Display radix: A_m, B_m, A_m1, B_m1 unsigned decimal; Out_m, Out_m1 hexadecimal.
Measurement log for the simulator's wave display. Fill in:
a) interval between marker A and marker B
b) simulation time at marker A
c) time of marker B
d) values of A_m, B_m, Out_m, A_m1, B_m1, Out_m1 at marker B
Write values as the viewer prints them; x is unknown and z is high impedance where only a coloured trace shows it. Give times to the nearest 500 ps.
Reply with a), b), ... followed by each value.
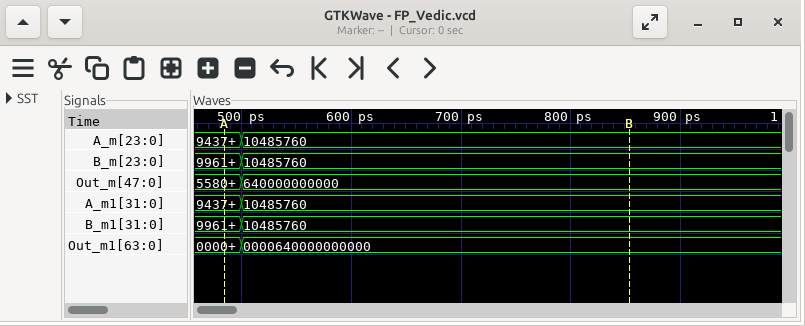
a) 500 ps
b) 500 ps
c) 1000 ps
d) A_m=10485760, B_m=10485760, Out_m=640000000000, A_m1=10485760, B_m1=10485760, Out_m1=0000640000000000
